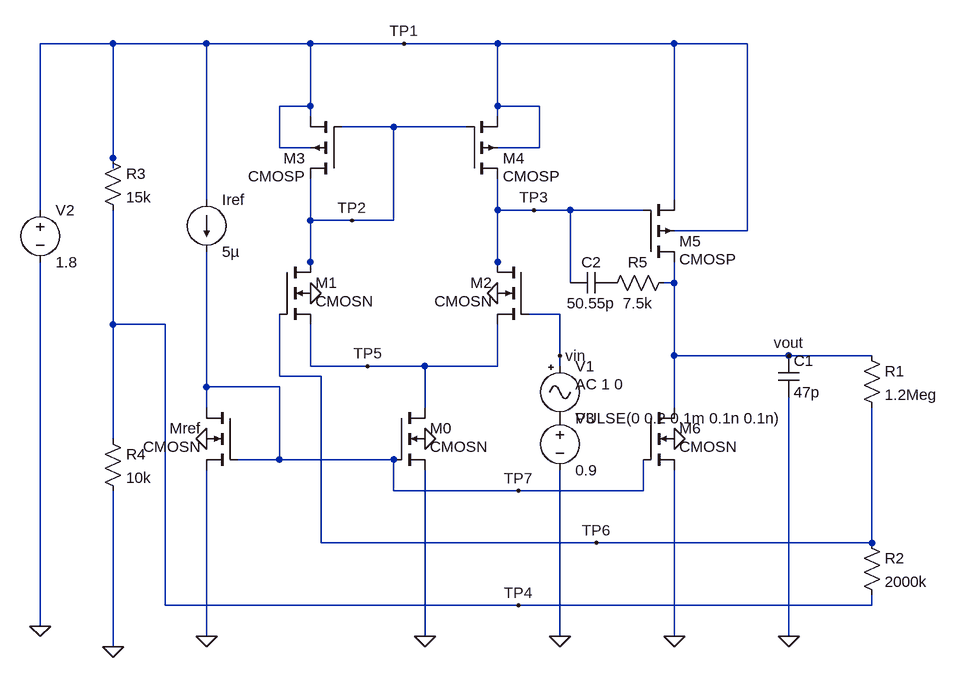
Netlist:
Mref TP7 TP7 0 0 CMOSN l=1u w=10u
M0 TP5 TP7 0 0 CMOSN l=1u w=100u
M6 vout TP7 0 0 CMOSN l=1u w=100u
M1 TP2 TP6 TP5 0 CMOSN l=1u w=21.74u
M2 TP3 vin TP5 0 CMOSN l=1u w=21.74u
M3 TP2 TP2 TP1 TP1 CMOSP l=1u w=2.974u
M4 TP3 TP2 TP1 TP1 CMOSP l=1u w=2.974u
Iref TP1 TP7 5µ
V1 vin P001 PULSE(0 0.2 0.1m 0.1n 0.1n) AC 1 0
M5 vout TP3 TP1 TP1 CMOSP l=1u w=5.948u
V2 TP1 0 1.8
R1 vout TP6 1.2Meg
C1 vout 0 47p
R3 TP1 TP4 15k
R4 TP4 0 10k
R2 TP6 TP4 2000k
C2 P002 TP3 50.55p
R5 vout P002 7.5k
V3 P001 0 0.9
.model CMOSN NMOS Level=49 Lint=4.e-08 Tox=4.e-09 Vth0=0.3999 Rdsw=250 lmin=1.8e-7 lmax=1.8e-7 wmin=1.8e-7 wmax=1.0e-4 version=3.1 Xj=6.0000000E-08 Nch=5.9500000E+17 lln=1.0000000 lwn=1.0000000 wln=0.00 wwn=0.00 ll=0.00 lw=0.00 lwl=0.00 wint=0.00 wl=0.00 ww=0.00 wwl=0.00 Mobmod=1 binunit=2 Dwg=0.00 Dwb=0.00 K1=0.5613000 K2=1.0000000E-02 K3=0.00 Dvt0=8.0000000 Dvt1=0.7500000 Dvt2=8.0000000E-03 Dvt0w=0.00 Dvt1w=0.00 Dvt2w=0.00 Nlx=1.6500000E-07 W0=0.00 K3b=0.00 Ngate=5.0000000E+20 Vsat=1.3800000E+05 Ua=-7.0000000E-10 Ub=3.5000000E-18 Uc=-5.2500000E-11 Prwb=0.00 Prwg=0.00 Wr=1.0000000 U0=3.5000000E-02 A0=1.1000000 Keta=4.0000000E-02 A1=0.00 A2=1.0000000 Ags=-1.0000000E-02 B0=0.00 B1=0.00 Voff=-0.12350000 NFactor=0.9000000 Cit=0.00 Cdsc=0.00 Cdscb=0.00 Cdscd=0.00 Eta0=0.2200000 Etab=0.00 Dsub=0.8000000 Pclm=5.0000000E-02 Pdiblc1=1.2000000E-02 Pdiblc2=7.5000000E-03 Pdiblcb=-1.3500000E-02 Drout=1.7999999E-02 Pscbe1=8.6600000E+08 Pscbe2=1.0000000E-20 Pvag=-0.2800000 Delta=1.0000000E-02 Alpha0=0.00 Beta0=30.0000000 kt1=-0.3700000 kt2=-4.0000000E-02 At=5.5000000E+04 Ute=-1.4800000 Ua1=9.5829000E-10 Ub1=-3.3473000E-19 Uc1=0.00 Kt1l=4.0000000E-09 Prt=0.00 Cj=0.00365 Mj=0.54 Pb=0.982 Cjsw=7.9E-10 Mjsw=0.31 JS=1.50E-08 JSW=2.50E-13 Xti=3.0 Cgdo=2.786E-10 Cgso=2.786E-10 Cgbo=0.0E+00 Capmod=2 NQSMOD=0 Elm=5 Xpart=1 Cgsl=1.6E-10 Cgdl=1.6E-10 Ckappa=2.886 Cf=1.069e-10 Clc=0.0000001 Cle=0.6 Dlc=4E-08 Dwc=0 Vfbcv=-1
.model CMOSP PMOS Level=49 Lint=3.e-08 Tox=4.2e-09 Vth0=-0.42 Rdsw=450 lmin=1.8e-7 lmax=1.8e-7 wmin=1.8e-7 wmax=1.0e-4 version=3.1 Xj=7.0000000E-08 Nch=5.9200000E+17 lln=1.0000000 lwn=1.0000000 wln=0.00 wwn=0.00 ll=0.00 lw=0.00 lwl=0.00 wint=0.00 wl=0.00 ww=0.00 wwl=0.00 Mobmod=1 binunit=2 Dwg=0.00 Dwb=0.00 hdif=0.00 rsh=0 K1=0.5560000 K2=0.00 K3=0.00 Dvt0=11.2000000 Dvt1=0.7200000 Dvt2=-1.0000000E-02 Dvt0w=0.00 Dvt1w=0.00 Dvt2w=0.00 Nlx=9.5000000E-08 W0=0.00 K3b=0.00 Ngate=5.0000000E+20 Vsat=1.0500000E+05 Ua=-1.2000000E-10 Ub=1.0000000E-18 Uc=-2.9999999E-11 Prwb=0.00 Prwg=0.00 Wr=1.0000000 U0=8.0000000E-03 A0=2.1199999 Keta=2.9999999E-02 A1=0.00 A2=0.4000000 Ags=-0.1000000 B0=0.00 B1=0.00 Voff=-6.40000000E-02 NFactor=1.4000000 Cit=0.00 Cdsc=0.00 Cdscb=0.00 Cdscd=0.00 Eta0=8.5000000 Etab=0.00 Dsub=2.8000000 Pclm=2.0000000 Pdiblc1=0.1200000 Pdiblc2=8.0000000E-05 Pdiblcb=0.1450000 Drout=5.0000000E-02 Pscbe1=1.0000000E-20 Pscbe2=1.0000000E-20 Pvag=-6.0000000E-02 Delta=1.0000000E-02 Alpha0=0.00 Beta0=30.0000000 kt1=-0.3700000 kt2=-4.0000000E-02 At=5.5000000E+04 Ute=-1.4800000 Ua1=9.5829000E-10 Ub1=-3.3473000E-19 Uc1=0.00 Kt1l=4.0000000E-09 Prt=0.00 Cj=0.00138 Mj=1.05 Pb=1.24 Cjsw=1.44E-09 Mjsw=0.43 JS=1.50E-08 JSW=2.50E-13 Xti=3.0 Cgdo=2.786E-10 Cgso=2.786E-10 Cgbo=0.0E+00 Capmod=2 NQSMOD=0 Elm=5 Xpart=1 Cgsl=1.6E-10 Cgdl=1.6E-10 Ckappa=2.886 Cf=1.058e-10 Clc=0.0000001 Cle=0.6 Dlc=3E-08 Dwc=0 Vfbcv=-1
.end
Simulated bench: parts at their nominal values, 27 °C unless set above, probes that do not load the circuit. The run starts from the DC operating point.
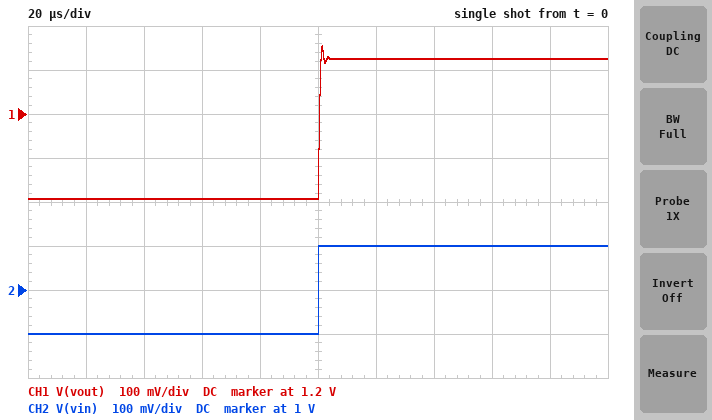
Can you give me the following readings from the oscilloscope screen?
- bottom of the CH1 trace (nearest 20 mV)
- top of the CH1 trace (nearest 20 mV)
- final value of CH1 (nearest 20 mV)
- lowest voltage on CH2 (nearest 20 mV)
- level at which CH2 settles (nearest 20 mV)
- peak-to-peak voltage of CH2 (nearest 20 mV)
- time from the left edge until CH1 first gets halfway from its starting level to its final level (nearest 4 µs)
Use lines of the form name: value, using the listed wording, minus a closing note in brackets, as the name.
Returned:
bottom of the CH1 trace: 1.00 V
top of the CH1 trace: 1.36 V
final value of CH1: 1.32 V
lowest voltage on CH2: 900 mV
level at which CH2 settles: 1.10 V
peak-to-peak voltage of CH2: 200 mV
time from the left edge until CH1 first gets halfway from its starting level to its final level: 100 µs
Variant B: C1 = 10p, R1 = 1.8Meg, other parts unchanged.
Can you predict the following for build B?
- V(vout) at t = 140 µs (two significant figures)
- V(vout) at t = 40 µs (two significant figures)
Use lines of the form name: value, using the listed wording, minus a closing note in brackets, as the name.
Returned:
V(vout) at t = 140 µs: 1.4 V
V(vout) at t = 40 µs: 1.1 V
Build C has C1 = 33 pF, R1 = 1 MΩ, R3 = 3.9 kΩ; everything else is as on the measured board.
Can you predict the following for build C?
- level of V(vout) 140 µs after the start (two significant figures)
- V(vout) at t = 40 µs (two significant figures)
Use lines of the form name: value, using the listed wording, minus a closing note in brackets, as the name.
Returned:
level of V(vout) 140 µs after the start: 1.0 V
V(vout) at t = 40 µs: 700 mV
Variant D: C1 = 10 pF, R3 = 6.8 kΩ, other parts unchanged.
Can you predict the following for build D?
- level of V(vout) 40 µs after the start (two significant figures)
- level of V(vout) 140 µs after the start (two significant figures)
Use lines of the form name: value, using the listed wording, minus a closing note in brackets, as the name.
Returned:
level of V(vout) 40 µs after the start: 800 mV
level of V(vout) 140 µs after the start: 1.1 V
